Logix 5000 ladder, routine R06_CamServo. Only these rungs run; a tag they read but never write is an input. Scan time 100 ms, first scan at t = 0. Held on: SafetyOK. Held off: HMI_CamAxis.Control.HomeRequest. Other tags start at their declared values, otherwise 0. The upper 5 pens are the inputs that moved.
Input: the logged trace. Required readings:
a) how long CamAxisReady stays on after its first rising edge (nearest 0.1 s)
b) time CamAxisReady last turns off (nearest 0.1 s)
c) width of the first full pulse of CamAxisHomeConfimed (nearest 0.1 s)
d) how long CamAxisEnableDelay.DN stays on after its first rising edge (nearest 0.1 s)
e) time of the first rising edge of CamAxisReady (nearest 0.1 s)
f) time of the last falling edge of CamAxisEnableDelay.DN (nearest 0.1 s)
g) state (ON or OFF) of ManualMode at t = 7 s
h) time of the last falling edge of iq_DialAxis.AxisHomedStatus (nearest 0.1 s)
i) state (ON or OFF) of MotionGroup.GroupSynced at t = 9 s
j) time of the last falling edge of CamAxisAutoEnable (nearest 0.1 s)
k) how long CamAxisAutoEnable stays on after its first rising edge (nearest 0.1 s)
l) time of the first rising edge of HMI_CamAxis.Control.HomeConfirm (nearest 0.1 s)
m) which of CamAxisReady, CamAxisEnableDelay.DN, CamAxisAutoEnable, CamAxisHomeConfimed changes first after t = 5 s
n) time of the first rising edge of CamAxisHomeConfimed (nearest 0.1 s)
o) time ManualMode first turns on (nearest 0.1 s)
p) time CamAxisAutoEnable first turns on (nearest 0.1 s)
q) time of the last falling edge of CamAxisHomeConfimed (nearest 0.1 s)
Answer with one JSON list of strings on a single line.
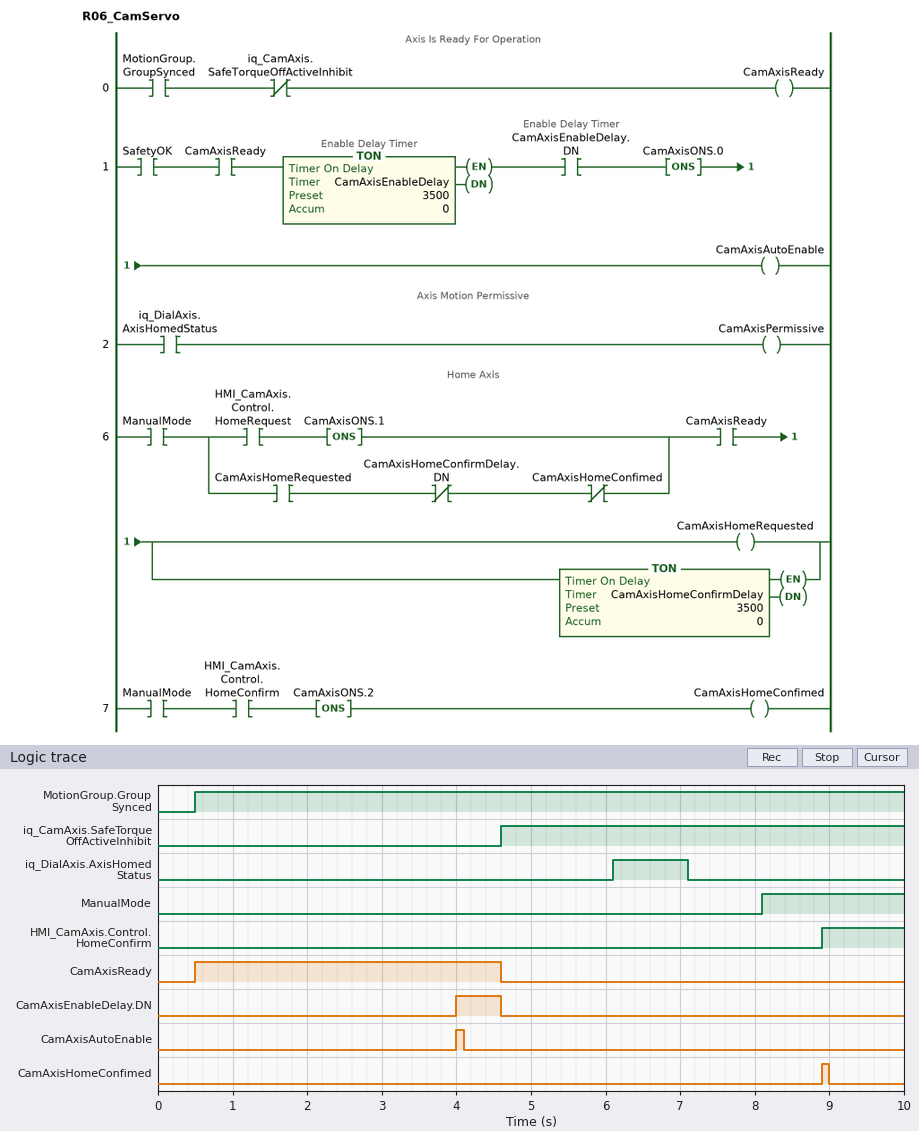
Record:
["4.1 s", "4.6 s", "0.1 s", "0.6 s", "0.5 s", "4.6 s", "OFF", "7.1 s", "ON", "4.1 s", "0.1 s", "8.9 s", "CamAxisHomeConfimed", "8.9 s", "8.1 s", "4.0 s", "9.0 s"]
